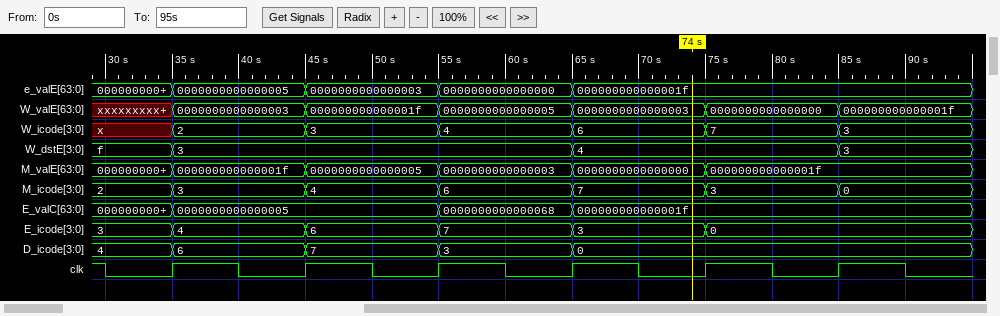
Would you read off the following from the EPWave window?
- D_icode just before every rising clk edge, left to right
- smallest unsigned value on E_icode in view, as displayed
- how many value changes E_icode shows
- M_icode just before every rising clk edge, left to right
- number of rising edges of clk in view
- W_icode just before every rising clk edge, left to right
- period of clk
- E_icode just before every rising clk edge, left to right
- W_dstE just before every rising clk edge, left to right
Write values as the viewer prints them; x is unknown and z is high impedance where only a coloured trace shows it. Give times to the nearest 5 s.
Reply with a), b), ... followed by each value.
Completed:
a) 4, 6, 7, 3, 0, 0
b) 0
c) 5
d) 2, 3, 4, 6, 7, 3
e) 6
f) x, 2, 3, 4, 6, 7
g) 10 s
h) 3, 4, 6, 7, 3, 0
i) f, 3, 3, 3, 4, 4
